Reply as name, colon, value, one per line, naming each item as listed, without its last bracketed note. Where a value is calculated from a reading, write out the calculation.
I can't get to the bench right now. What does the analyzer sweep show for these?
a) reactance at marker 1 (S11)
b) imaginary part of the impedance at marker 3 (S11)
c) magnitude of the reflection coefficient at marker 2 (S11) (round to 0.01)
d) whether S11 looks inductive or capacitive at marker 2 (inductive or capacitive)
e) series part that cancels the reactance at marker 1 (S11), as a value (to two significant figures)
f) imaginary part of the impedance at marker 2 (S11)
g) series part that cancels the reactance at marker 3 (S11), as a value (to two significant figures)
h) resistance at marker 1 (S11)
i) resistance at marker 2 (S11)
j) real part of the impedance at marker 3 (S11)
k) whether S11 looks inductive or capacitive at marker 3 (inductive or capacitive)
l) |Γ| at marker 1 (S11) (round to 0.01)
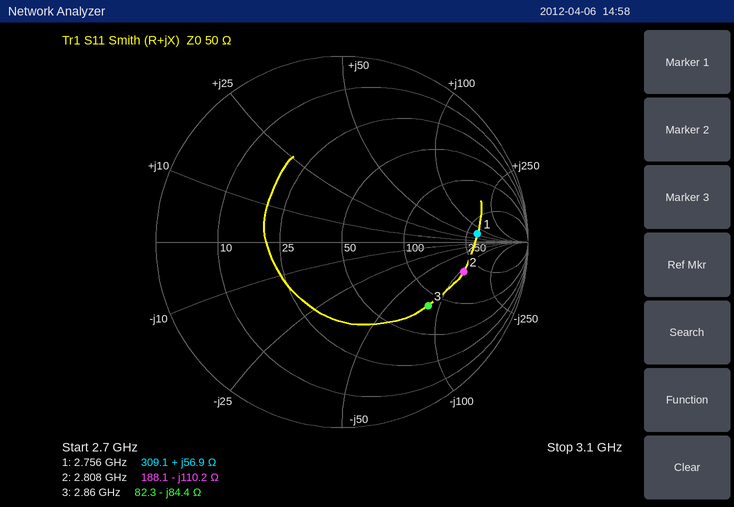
reactance at marker 1: +56.9 Ω
imaginary part of the impedance at marker 3: -84.4 Ω
magnitude of the reflection coefficient at marker 2 (S11): 0.67
whether S11 looks inductive or capacitive at marker 2: capacitive
series part that cancels the reactance at marker 1 (S11), as a value: C = 1/(2π × 2.756 GHz × 56.9 Ω) ≈ 1.0 pF
imaginary part of the impedance at marker 2: -110.2 Ω
series part that cancels the reactance at marker 3 (S11), as a value: L = 84.4 Ω/(2π × 2.86 GHz) ≈ 4.7 nH
resistance at marker 1: 309.1 Ω
resistance at marker 2: 188.1 Ω
real part of the impedance at marker 3: 82.3 Ω
whether S11 looks inductive or capacitive at marker 3: capacitive
|Γ| at marker 1 (S11): 0.73
